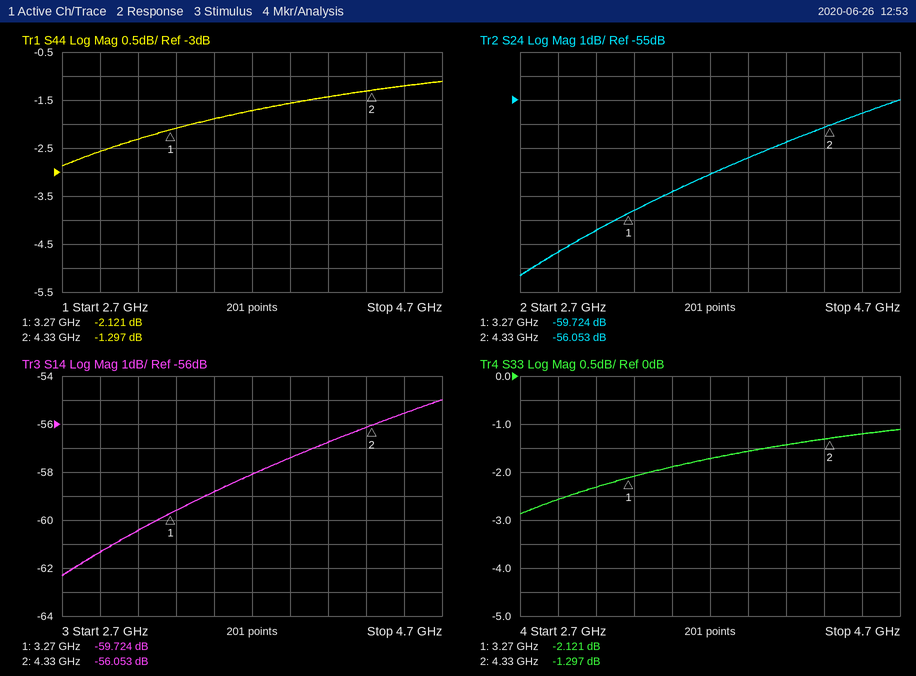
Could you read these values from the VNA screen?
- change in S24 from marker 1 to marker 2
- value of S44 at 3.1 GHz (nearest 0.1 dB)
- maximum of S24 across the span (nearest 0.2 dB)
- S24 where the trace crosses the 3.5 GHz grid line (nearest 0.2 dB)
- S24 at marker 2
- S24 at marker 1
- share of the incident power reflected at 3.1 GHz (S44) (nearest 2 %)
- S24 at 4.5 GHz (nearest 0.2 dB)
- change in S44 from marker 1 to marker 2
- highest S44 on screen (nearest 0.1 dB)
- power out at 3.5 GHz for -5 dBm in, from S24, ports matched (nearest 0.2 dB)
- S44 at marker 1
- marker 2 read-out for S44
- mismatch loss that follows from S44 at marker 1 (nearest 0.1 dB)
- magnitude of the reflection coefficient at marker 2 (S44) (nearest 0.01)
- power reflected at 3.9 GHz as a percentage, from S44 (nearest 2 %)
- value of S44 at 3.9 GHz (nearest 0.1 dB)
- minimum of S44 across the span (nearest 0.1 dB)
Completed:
3.671 dB
-2.3 dB
-55.0 dB
-58.8 dB
-56.053 dB
-59.724 dB
58 %
-55.6 dB
0.824 dB
-1.1 dB
-63.8 dBm
-2.121 dB
-1.297 dB
4.1 dB
0.86
70 %
-1.6 dB
-2.9 dB
